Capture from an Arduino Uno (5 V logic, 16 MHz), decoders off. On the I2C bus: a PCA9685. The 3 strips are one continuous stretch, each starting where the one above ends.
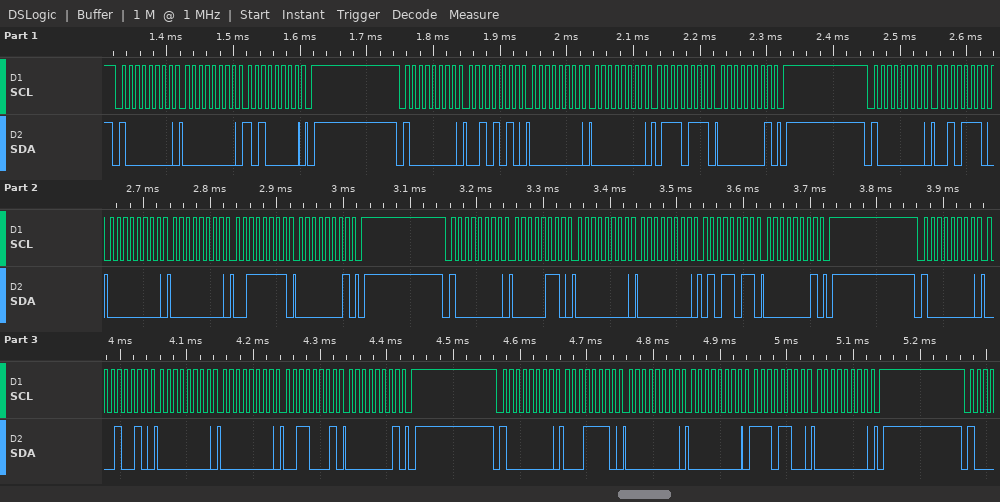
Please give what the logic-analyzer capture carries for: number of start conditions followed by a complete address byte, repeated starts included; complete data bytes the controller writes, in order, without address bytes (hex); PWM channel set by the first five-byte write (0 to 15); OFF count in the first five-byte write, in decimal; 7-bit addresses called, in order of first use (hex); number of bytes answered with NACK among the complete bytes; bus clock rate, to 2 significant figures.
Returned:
6
00 A0 2A 00 00 77 01 2E 00 00 3F 01 06 00 00 5B 01 12 00 00 31 01 1E 00 00 EC 00
9
375
0x40
0
100 kHz
